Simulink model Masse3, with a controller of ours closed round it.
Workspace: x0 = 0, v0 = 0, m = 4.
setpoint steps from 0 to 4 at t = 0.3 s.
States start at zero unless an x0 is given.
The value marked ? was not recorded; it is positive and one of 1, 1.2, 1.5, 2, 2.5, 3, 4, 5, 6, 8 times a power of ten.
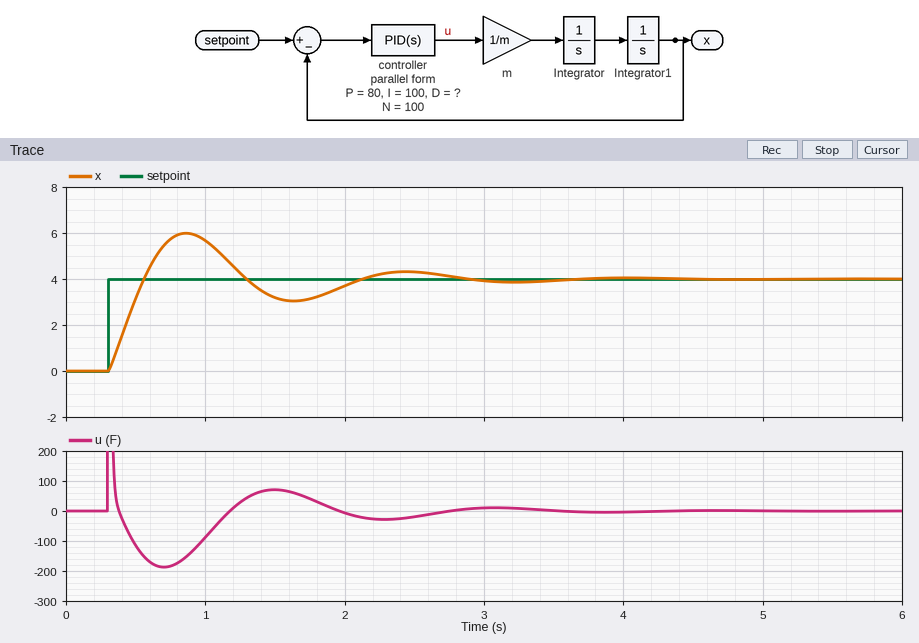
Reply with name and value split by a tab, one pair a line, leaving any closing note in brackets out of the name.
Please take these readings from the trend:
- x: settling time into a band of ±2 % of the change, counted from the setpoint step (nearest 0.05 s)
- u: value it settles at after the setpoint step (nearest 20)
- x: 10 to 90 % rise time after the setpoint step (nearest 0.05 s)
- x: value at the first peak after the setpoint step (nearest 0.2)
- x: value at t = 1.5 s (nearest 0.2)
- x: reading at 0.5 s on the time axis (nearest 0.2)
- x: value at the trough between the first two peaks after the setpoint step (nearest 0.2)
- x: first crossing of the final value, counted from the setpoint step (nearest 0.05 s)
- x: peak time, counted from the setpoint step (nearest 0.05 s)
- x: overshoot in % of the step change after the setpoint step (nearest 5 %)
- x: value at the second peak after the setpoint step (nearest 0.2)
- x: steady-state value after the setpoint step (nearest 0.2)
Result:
x: settling time into a band of ±2 % of the change, counted from the setpoint step	3.20 s
u: value it settles at after the setpoint step	0
x: 10 to 90 % rise time after the setpoint step	0.20 s
x: value at the first peak after the setpoint step	6.0
x: value at t = 1.5 s	3.2
x: reading at 0.5 s on the time axis	3.2
x: value at the trough between the first two peaks after the setpoint step	3.0
x: first crossing of the final value, counted from the setpoint step	0.25 s
x: peak time, counted from the setpoint step	0.55 s
x: overshoot in % of the step change after the setpoint step	50 %
x: value at the second peak after the setpoint step	4.4
x: steady-state value after the setpoint step	4.0
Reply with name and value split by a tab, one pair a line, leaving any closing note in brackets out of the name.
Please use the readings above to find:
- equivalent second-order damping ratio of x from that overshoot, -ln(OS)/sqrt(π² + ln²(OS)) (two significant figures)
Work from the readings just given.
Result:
equivalent second-order damping ratio of x from that overshoot, -ln(OS)/sqrt(π² + ln²(OS))	0.22
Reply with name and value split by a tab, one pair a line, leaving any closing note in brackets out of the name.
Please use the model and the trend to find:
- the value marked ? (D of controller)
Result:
the value marked ?	15
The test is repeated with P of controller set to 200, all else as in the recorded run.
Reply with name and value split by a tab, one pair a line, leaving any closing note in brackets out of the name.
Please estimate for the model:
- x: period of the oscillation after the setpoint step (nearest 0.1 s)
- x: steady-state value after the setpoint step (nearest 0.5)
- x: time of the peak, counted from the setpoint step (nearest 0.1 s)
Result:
x: period of the oscillation after the setpoint step	0.9 s
x: steady-state value after the setpoint step	4.0
x: time of the peak, counted from the setpoint step	0.4 s
